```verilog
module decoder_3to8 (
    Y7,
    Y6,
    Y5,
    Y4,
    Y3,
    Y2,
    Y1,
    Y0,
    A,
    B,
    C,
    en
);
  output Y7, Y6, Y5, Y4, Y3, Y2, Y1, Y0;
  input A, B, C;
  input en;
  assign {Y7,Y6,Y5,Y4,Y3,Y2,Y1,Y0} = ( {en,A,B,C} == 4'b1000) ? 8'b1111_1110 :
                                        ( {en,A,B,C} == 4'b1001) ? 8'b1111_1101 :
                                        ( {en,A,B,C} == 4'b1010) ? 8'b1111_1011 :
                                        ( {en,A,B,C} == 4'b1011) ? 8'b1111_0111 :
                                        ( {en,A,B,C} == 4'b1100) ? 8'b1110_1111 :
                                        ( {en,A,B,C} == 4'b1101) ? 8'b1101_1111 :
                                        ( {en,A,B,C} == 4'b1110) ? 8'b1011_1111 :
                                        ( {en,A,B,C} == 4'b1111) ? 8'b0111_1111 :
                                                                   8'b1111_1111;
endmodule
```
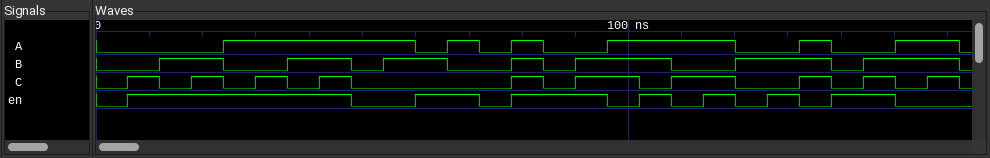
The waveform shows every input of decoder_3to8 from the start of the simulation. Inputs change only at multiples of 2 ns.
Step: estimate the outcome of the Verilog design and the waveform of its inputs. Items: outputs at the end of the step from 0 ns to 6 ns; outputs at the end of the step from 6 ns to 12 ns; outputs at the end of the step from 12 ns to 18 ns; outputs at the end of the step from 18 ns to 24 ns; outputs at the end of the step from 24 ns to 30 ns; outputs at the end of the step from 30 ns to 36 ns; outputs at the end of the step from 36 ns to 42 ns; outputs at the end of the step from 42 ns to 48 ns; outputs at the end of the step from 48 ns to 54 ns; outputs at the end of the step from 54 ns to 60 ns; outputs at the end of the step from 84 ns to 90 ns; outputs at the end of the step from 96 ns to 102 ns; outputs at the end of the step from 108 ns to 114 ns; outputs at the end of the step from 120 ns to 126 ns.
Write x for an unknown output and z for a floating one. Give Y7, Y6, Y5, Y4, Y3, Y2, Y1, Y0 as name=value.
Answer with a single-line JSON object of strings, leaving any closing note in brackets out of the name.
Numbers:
{"outputs at the end of the step from 0 ns to 6 ns": "Y7=1, Y6=1, Y5=1, Y4=1, Y3=1, Y2=1, Y1=1, Y0=1", "outputs at the end of the step from 6 ns to 12 ns": "Y7=1, Y6=1, Y5=1, Y4=1, Y3=1, Y2=1, Y1=0, Y0=1", "outputs at the end of the step from 12 ns to 18 ns": "Y7=1, Y6=1, Y5=1, Y4=1, Y3=1, Y2=0, Y1=1, Y0=1", "outputs at the end of the step from 18 ns to 24 ns": "Y7=1, Y6=1, Y5=1, Y4=1, Y3=0, Y2=1, Y1=1, Y0=1", "outputs at the end of the step from 24 ns to 30 ns": "Y7=1, Y6=1, Y5=1, Y4=0, Y3=1, Y2=1, Y1=1, Y0=1", "outputs at the end of the step from 30 ns to 36 ns": "Y7=1, Y6=1, Y5=0, Y4=1, Y3=1, Y2=1, Y1=1, Y0=1", "outputs at the end of the step from 36 ns to 42 ns": "Y7=1, Y6=0, Y5=1, Y4=1, Y3=1, Y2=1, Y1=1, Y0=1", "outputs at the end of the step from 42 ns to 48 ns": "Y7=0, Y6=1, Y5=1, Y4=1, Y3=1, Y2=1, Y1=1, Y0=1", "outputs at the end of the step from 48 ns to 54 ns": "Y7=1, Y6=1, Y5=1, Y4=1, Y3=1, Y2=1, Y1=1, Y0=1", "outputs at the end of the step from 54 ns to 60 ns": "Y7=1, Y6=1, Y5=1, Y4=1, Y3=1, Y2=1, Y1=1, Y0=1", "outputs at the end of the step from 84 ns to 90 ns": "Y7=1, Y6=1, Y5=1, Y4=1, Y3=1, Y2=1, Y1=1, Y0=0", "outputs at the end of the step from 96 ns to 102 ns": "Y7=1, Y6=1, Y5=1, Y4=1, Y3=1, Y2=1, Y1=1, Y0=1", "outputs at the end of the step from 108 ns to 114 ns": "Y7=1, Y6=1, Y5=1, Y4=1, Y3=1, Y2=1, Y1=1, Y0=1", "outputs at the end of the step from 120 ns to 126 ns": "Y7=1, Y6=1, Y5=1, Y4=1, Y3=1, Y2=1, Y1=1, Y0=1"}
